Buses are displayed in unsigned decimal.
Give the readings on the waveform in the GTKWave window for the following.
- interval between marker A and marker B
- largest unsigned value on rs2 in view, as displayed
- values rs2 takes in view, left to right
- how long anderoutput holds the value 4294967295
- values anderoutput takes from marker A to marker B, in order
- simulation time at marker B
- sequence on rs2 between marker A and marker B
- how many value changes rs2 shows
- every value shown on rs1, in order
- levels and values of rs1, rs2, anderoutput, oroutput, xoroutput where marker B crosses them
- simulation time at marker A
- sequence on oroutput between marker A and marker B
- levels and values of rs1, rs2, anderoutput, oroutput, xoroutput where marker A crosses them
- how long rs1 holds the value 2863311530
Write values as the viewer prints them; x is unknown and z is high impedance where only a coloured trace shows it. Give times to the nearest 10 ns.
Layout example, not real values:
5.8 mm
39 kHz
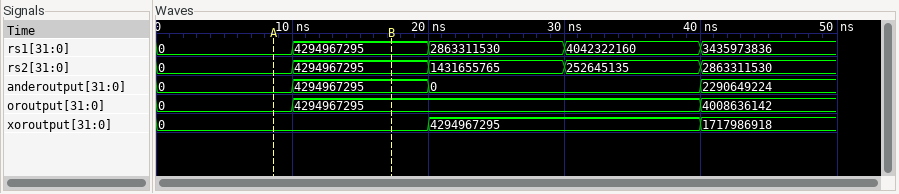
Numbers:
10 ns
4294967295
0, 4294967295, 1431655765, 252645135, 2863311530
10 ns
0, 4294967295
20 ns
0, 4294967295
4
0, 4294967295, 2863311530, 4042322160, 3435973836
rs1=4294967295, rs2=4294967295, anderoutput=4294967295, oroutput=4294967295, xoroutput=0
10 ns
0, 4294967295
rs1=0, rs2=0, anderoutput=0, oroutput=0, xoroutput=0
10 ns
